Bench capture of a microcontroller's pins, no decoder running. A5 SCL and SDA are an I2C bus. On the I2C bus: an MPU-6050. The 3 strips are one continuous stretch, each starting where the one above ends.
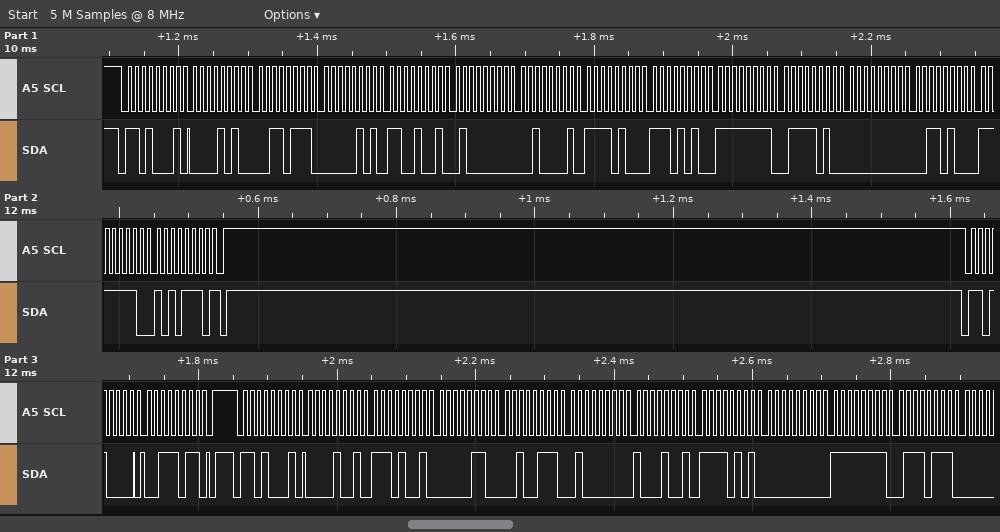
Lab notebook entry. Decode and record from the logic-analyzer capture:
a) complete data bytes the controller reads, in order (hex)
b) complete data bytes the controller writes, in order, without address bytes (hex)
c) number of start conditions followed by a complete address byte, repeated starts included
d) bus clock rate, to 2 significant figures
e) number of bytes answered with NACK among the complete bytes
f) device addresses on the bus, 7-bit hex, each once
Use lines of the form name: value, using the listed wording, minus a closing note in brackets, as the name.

complete data bytes the controller reads, in order: 0A 37 05 C9 40 21 F4 EA FF 7A 00 34 FE AE 09 E9 06 27 40 89 F5 00 FF 77
complete data bytes the controller writes, in order, without address bytes: 3B
number of start conditions followed by a complete address byte, repeated starts included: 3
bus clock rate, to 2 significant figures: 100 kHz
number of bytes answered with NACK among the complete bytes: 1
device addresses on the bus, 7-bit hex, each once: 0x68
